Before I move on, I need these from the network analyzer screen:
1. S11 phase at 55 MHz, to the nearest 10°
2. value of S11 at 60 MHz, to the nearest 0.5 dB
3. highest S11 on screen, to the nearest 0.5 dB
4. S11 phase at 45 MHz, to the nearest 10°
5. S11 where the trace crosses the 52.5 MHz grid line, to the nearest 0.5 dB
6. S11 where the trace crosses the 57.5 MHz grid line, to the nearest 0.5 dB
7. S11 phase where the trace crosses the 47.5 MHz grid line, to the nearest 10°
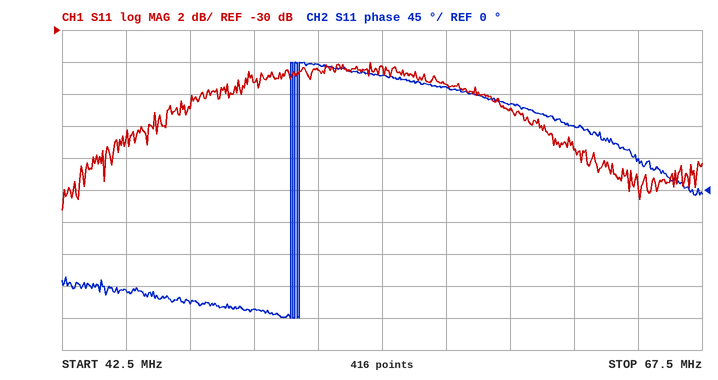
160°
-35.0 dB
-32.0 dB
-140°
-32.5 dB
-33.5 dB
-160°
